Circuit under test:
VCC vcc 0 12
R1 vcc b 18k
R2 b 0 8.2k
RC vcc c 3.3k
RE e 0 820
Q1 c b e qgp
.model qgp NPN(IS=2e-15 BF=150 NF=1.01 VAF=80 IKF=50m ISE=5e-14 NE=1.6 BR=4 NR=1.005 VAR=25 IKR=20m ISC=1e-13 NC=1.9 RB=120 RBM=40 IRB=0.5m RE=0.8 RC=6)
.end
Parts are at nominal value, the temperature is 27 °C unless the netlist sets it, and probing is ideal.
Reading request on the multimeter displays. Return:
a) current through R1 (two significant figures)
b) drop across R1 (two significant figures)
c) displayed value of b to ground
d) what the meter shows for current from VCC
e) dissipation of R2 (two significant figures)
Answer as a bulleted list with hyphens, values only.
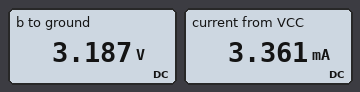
- 490 µA
- 8.8 V
- 3.187 V
- 3.361 mA
- 1.2 mW
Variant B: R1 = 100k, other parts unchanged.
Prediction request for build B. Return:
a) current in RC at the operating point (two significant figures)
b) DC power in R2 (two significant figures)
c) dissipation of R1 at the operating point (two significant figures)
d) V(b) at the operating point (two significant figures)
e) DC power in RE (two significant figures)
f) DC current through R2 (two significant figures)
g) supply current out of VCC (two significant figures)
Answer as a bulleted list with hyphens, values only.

- 270 µA
- 97 µW
- 1.2 mW
- 890 mV
- 62 µW
- 110 µA
- 380 µA
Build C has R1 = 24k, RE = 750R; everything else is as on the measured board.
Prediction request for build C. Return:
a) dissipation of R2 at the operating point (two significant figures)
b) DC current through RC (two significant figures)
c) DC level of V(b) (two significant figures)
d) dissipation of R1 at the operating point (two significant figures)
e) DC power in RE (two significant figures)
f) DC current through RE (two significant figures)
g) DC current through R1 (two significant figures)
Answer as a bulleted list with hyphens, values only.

- 1.0 mW
- 2.9 mA
- 2.9 V
- 3.4 mW
- 6.3 mW
- 2.9 mA
- 380 µA
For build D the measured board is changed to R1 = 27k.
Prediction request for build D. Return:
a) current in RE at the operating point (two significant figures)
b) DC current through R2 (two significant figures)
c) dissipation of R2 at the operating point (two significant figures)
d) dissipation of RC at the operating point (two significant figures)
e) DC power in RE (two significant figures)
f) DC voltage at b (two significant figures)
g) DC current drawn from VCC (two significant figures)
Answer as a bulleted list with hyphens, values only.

- 2.4 mA
- 330 µA
- 870 µW
- 18 mW
- 4.6 mW
- 2.7 V
- 2.7 mA
